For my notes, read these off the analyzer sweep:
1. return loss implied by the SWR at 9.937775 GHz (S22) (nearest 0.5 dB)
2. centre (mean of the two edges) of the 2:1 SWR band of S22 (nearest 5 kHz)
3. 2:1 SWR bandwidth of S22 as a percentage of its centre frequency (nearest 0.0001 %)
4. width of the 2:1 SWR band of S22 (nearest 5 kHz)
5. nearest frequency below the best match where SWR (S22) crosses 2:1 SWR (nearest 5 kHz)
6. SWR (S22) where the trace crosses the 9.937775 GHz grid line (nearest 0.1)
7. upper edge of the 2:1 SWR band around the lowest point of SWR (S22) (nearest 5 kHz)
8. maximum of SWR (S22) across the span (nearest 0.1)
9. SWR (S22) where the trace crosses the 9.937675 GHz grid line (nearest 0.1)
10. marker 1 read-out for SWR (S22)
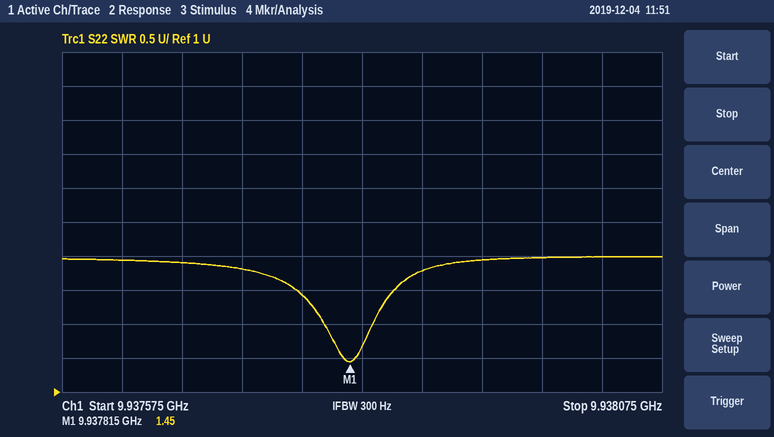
7.5 dB
9.937815 GHz
0.0004 %
40 kHz
9.937795 GHz
2.4
9.937835 GHz
3.0
2.9
1.45
